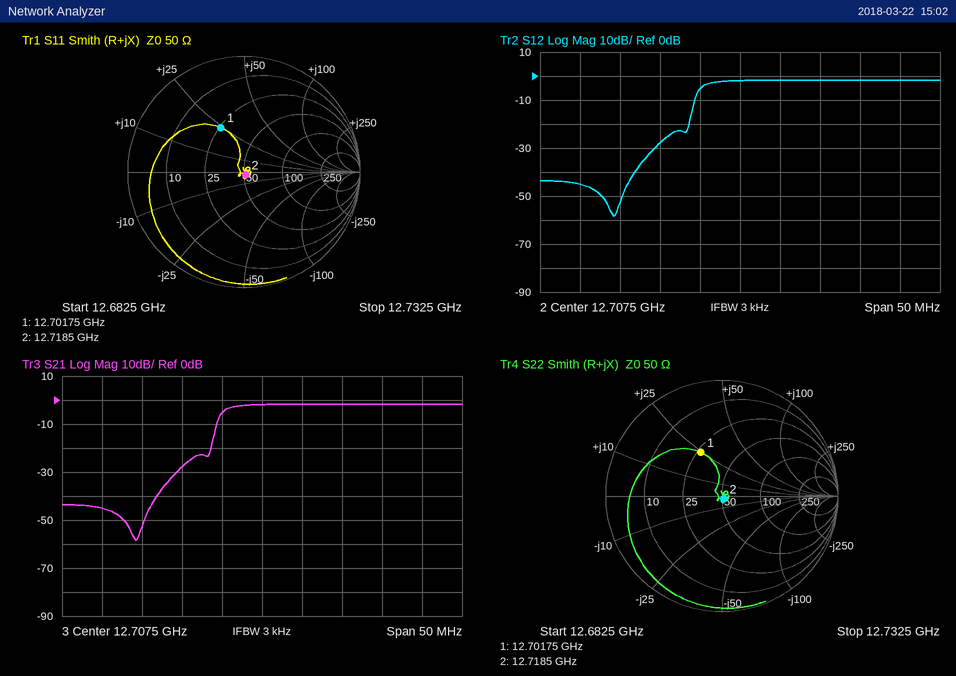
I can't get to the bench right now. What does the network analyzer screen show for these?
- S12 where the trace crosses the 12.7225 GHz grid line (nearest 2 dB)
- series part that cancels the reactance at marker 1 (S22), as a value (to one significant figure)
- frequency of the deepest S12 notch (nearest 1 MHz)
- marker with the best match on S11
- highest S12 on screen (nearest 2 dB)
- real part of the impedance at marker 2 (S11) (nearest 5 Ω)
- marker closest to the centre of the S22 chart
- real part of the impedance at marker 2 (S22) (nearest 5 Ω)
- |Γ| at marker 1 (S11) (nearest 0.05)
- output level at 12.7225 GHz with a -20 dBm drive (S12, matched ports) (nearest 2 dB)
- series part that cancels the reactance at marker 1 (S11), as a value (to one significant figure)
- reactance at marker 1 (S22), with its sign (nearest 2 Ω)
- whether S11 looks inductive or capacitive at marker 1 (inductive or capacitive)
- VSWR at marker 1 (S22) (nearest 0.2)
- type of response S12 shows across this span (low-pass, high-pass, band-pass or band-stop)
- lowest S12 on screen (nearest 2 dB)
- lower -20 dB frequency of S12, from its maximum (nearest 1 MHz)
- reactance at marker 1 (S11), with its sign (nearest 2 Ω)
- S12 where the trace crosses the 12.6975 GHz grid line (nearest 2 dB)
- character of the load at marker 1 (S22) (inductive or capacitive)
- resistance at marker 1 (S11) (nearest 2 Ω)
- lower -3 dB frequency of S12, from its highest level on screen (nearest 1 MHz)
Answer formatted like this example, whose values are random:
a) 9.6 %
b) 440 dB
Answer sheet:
a) -2 dB
b) 500 fF
c) 12.692 GHz
d) marker 2
e) -2 dB
f) 50 Ω
g) marker 2
h) 50 Ω
i) 0.45
j) -22 dBm
k) 500 fF
l) +24 Ω
m) inductive
n) 2.4
o) high-pass
p) -58 dB
q) 12.701 GHz
r) +24 Ω
s) -28 dB
t) inductive
u) 26 Ω
v) 12.703 GHz
